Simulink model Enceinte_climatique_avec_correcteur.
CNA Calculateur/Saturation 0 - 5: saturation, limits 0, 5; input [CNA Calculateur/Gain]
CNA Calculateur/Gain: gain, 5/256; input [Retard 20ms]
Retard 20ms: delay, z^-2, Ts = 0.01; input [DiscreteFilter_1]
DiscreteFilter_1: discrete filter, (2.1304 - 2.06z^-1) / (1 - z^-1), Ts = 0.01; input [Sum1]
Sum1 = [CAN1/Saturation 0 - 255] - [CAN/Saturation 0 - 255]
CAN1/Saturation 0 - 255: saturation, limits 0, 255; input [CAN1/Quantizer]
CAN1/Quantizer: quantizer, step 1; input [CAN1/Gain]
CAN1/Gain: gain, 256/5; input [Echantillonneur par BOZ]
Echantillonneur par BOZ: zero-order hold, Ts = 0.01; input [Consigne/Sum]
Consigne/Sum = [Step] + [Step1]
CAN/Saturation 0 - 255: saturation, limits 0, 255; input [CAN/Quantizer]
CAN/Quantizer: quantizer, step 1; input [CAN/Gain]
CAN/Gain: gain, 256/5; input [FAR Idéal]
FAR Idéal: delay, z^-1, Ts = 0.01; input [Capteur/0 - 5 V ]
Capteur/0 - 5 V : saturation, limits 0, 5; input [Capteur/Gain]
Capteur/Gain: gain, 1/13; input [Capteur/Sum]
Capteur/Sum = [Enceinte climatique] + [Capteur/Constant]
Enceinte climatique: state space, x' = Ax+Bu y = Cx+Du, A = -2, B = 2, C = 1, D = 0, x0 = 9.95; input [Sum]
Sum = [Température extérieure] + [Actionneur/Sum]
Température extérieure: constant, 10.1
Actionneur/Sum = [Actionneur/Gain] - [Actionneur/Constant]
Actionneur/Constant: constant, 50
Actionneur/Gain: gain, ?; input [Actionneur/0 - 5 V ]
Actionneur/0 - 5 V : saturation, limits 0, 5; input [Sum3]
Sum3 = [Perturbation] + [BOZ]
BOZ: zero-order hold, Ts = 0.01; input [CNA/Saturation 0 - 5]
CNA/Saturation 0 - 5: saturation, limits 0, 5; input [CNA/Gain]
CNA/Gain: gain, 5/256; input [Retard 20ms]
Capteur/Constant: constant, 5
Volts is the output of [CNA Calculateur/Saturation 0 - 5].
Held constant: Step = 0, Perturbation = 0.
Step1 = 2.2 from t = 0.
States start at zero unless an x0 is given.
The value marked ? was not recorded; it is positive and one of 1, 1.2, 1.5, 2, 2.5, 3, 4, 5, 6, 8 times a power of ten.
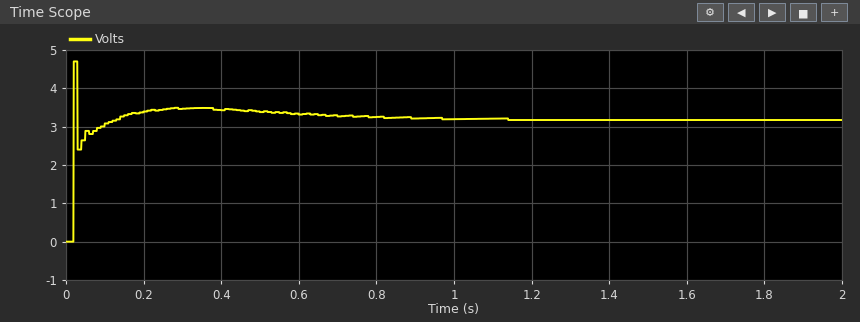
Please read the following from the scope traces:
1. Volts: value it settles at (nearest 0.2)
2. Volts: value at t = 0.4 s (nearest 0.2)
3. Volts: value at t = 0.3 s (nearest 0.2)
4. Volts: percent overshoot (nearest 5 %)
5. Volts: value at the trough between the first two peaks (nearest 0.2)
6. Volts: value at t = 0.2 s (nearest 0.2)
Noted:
3.2
3.4
3.4
50 %
2.4
3.4
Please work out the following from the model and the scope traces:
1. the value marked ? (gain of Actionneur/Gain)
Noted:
20
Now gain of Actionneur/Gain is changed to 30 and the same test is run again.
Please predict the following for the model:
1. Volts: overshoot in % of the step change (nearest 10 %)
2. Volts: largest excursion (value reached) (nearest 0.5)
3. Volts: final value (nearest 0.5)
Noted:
120 %
4.5
2.0
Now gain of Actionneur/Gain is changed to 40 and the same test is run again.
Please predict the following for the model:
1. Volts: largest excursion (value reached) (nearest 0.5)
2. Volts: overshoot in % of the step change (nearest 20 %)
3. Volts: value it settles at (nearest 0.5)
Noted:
4.5
200 %
1.5
